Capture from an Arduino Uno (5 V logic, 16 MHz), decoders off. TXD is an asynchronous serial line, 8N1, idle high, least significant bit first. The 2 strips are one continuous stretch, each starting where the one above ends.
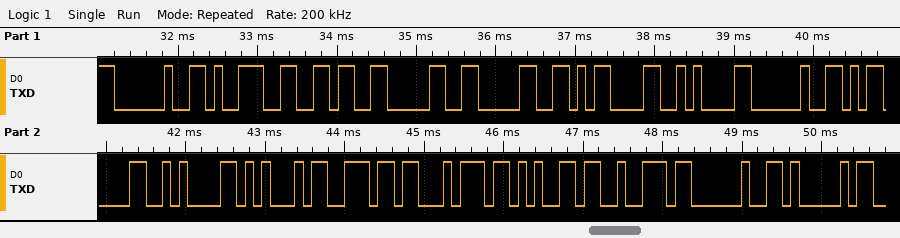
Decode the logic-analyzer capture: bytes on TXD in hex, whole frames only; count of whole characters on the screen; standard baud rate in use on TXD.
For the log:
20 39 36 30 30 0D 0A 20 0D 0A 45 6E 74 65 72 20 41
17
9600 baud
